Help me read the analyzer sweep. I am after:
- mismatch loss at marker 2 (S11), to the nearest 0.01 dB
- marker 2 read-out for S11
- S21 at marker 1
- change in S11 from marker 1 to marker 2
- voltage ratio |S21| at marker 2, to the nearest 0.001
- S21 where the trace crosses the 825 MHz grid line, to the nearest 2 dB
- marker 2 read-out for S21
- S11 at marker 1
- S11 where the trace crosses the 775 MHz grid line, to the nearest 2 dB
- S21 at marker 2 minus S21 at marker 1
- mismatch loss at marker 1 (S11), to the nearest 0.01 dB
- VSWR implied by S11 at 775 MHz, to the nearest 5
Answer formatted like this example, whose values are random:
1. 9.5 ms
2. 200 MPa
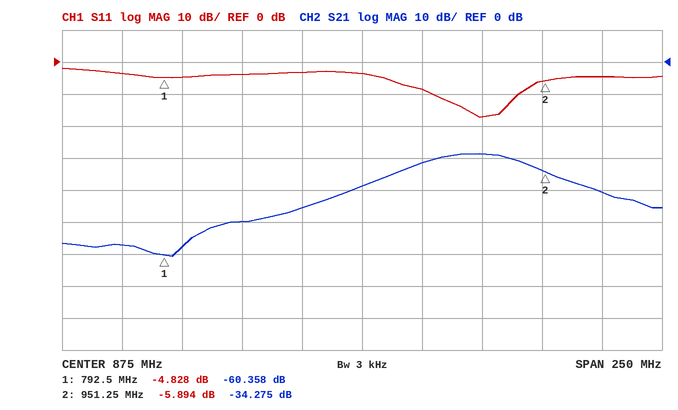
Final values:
1. 1.29 dB
2. -5.894 dB
3. -60.358 dB
4. -1.066 dB
5. 0.019
6. -50 dB
7. -34.275 dB
8. -4.828 dB
9. -4 dB
10. 26.083 dB
11. 1.73 dB
12. 5
